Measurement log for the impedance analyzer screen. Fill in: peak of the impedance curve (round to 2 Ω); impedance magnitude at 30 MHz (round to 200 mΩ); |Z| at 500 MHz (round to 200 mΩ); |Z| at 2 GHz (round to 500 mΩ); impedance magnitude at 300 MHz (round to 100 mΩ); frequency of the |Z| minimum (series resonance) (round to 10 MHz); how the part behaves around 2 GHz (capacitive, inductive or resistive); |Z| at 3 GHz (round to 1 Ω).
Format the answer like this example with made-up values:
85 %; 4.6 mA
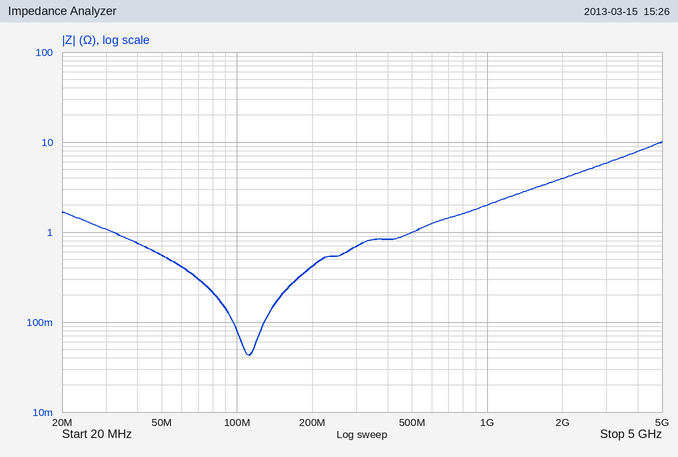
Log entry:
10 Ω; 1.0 Ω; 1.0 Ω; 4.0 Ω; 700 mΩ; 110 MHz; inductive; 6 Ω
